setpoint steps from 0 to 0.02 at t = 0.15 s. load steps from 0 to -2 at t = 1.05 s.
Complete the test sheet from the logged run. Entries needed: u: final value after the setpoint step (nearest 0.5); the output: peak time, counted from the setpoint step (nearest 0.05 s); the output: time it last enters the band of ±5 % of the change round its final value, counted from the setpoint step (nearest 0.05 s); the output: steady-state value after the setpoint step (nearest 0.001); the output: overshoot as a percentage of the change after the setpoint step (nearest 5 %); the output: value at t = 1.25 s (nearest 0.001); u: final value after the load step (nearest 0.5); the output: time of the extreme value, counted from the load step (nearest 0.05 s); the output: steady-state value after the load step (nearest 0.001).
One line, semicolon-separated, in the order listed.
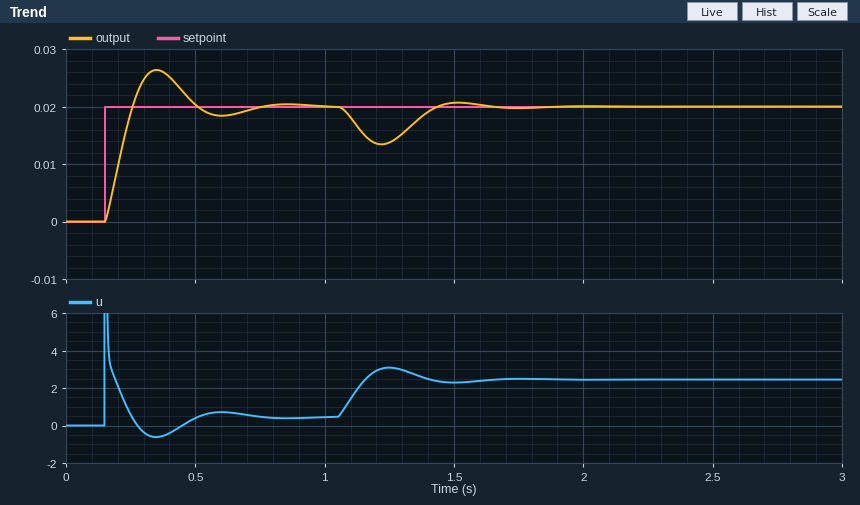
0.5; 0.20 s; 0.55 s; 0.020; 30 %; 0.014; 2.5; 0.15 s; 0.020
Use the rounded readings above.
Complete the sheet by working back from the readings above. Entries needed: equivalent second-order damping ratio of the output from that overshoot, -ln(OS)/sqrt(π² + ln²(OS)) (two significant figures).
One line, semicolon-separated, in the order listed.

0.36
